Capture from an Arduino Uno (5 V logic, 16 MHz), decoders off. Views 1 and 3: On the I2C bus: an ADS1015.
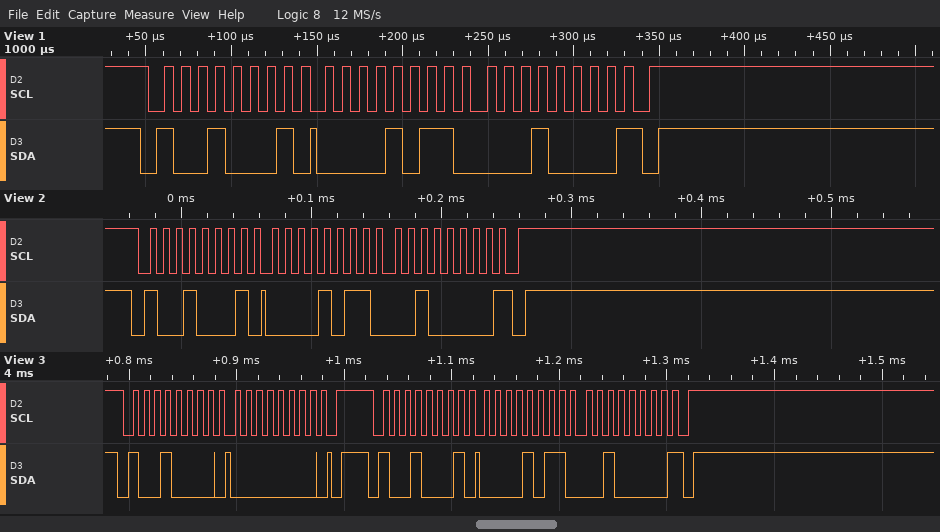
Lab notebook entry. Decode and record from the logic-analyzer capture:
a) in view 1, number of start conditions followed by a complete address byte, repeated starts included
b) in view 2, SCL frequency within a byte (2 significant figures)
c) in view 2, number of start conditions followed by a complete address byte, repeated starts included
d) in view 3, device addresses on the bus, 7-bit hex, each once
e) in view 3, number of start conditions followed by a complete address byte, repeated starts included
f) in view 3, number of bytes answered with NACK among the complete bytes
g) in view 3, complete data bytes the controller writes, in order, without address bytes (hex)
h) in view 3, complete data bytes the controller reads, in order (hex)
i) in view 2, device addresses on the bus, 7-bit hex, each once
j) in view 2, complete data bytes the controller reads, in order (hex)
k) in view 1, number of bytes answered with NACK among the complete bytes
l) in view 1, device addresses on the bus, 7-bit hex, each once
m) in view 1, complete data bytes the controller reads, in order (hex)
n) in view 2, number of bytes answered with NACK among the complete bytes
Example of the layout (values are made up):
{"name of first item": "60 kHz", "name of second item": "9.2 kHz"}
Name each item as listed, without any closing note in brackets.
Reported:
{"in view 1, number of start conditions followed by a complete address byte, repeated starts included": "1", "in view 2, SCL frequency within a byte": "100 kHz", "in view 2, number of start conditions followed by a complete address byte, repeated starts included": "1", "in view 3, device addresses on the bus, 7-bit hex, each once": "0x48", "in view 3, number of start conditions followed by a complete address byte, repeated starts included": "2", "in view 3, number of bytes answered with NACK among the complete bytes": "1", "in view 3, complete data bytes the controller writes, in order, without address bytes": "00", "in view 3, complete data bytes the controller reads, in order": "0B 20", "in view 2, device addresses on the bus, 7-bit hex, each once": "0x48", "in view 2, complete data bytes the controller reads, in order": "0B 20", "in view 1, number of bytes answered with NACK among the complete bytes": "1", "in view 1, device addresses on the bus, 7-bit hex, each once": "0x48", "in view 1, complete data bytes the controller reads, in order": "0B 10", "in view 2, number of bytes answered with NACK among the complete bytes": "1"}
